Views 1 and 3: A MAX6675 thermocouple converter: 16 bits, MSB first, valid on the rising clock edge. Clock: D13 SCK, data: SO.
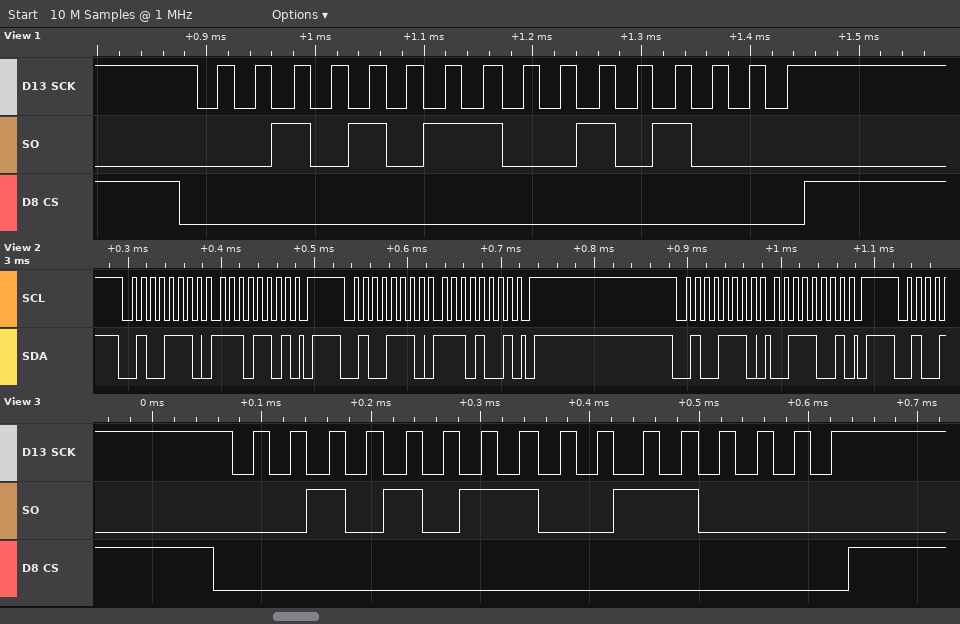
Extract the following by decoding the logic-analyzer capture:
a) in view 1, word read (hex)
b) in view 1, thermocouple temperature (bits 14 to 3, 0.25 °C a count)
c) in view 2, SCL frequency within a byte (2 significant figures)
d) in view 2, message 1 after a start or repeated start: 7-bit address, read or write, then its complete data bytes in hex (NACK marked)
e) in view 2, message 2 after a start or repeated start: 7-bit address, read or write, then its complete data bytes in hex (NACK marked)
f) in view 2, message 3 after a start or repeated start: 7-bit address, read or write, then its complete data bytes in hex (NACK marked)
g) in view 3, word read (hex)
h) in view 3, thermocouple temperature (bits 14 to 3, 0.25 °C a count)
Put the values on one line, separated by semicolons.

0x2B28; 345.25 °C; 100 kHz; 0x27 write: ED; 0x27 write: E9; 0x27 write: 39; 0x2B30; 345.50 °C
